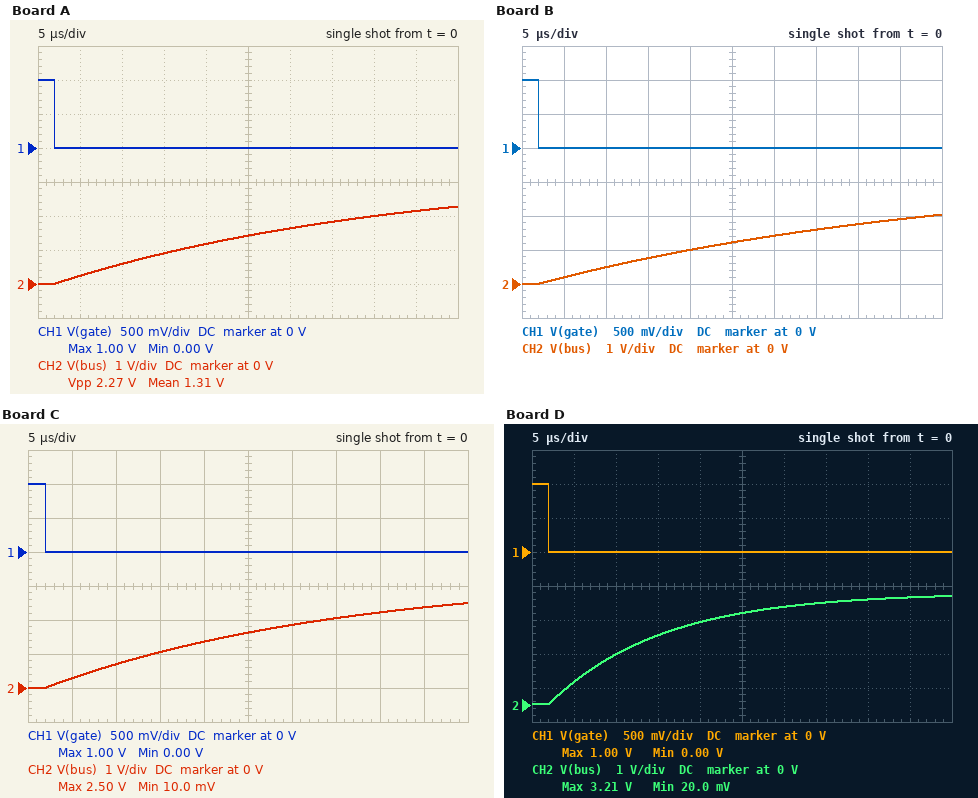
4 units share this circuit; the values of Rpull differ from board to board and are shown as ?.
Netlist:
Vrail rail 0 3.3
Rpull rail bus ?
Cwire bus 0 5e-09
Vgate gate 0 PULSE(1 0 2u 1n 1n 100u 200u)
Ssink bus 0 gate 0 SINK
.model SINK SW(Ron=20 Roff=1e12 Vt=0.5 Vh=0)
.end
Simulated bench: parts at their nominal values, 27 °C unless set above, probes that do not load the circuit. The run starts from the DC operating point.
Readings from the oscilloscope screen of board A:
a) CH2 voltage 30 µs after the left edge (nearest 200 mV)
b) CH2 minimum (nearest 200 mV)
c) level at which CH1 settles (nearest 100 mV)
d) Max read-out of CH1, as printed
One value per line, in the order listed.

1.6 V
0 V
0 V
1.00 V
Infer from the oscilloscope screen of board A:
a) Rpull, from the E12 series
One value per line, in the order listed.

8.2 kΩ
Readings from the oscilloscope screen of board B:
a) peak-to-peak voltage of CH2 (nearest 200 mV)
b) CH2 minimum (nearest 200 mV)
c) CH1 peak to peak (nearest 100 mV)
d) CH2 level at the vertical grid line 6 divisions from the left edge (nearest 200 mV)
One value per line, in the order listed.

2.0 V
0 V
1.0 V
1.4 V
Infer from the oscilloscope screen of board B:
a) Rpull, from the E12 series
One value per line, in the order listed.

10 kΩ
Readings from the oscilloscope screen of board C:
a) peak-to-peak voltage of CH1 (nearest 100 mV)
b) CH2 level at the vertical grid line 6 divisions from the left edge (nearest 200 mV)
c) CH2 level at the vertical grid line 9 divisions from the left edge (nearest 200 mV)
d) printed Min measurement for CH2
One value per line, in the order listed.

1.0 V
1.8 V
2.4 V
10.0 mV
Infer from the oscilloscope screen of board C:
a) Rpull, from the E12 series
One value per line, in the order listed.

6.8 kΩ
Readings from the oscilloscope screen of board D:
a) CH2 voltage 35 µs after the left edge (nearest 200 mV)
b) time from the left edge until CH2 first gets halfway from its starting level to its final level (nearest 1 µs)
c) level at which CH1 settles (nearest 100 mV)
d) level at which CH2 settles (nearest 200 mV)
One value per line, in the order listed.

3.0 V
11 µs
0 V
3.2 V
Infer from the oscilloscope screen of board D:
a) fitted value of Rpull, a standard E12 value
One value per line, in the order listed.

2.7 kΩ
